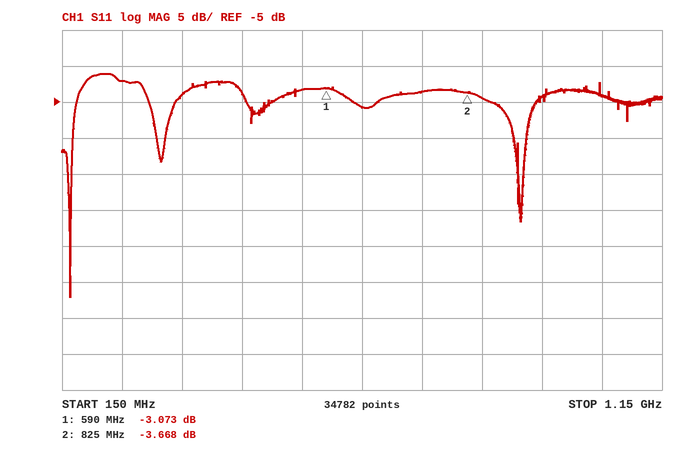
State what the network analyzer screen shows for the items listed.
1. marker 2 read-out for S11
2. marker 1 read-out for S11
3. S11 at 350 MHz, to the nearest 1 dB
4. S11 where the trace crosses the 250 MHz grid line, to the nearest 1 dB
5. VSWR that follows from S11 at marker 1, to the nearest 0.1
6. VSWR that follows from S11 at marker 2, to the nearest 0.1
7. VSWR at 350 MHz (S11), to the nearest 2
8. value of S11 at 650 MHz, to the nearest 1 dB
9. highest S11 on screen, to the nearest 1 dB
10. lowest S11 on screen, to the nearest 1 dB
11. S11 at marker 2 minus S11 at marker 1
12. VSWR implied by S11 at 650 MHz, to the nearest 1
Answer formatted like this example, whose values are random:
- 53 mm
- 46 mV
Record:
- -3.668 dB
- -3.073 dB
- -4 dB
- -2 dB
- 5.7
- 4.8
- 4
- -6 dB
- -1 dB
- -32 dB
- -0.595 dB
- 3
